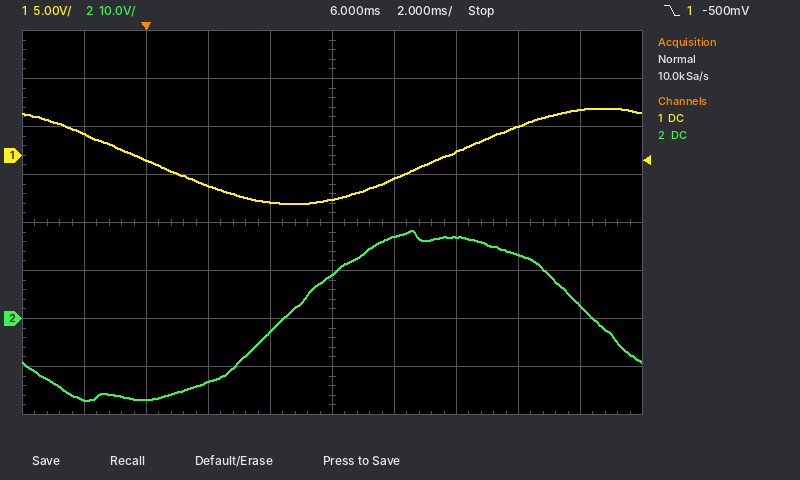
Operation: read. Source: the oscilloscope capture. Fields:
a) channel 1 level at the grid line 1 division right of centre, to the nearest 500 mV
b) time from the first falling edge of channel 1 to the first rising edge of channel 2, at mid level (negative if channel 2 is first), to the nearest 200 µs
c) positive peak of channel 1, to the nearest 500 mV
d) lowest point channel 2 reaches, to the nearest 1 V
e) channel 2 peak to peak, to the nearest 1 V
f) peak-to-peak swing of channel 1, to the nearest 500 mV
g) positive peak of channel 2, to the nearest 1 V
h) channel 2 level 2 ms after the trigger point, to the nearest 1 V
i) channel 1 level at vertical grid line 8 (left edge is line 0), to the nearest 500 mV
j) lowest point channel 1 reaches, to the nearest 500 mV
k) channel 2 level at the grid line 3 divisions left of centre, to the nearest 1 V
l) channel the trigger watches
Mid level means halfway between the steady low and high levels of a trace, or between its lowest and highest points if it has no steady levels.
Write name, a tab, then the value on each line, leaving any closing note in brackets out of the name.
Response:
channel 1 level at the grid line 1 division right of centre, to the nearest 500 mV	-2.5 V
time from the first falling edge of channel 1 to the first rising edge of channel 2, at mid level (negative if channel 2 is first), to the nearest 200 µs	+4.8 ms
positive peak of channel 1, to the nearest 500 mV	5.0 V
lowest point channel 2 reaches, to the nearest 1 V	-17 V
channel 2 peak to peak, to the nearest 1 V	35 V
peak-to-peak swing of channel 1, to the nearest 500 mV	10.0 V
positive peak of channel 2, to the nearest 1 V	18 V
channel 2 level 2 ms after the trigger point, to the nearest 1 V	-13 V
channel 1 level at vertical grid line 8 (left edge is line 0), to the nearest 500 mV	3.0 V
lowest point channel 1 reaches, to the nearest 500 mV	-5.0 V
channel 2 level at the grid line 3 divisions left of centre, to the nearest 1 V	-17 V
channel the trigger watches	channel 1
